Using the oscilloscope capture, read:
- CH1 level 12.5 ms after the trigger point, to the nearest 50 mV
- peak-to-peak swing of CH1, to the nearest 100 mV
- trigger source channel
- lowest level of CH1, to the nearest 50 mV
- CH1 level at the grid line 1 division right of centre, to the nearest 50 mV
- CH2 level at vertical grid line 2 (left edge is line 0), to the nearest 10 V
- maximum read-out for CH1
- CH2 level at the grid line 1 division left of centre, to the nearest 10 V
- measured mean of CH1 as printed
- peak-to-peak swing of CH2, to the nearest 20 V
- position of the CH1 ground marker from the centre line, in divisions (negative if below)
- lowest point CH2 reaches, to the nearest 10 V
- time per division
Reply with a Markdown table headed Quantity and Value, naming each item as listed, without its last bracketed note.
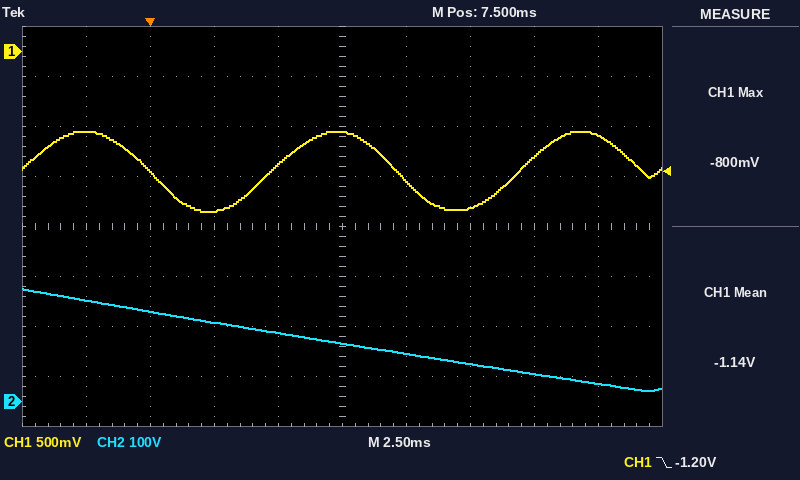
| Quantity | Value |
|---|---|
| CH1 level 12.5 ms after the trigger point, to the nearest 50 mV | -1.55 V |
| peak-to-peak swing of CH1, to the nearest 100 mV | 800 mV |
| trigger source channel | CH1 |
| lowest level of CH1, to the nearest 50 mV | -1.60 V |
| CH1 level at the grid line 1 division right of centre, to the nearest 50 mV | -1.30 V |
| CH2 level at vertical grid line 2 (left edge is line 0), to the nearest 10 V | 180 V |
| maximum read-out for CH1 | -800 mV |
| CH2 level at the grid line 1 division left of centre, to the nearest 10 V | 140 V |
| measured mean of CH1 as printed | -1.14 V |
| peak-to-peak swing of CH2, to the nearest 20 V | 200 V |
| position of the CH1 ground marker from the centre line, in divisions | +3.5 div |
| lowest point CH2 reaches, to the nearest 10 V | 20 V |
| time per division | 2.5 ms |
